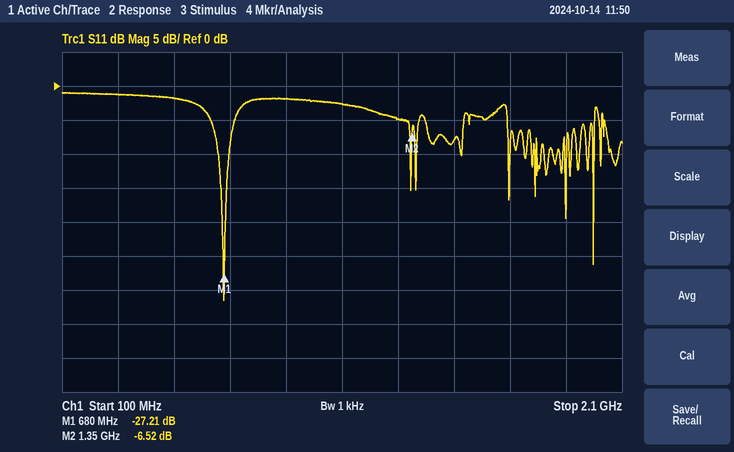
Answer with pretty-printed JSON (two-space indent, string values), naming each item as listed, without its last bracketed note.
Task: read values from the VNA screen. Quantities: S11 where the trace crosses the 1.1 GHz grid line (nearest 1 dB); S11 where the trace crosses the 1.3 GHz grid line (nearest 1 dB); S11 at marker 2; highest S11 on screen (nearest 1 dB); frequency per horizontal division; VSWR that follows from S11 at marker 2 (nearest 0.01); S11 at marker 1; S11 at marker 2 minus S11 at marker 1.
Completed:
{
  "S11 where the trace crosses the 1.1 GHz grid line": "-3 dB",
  "S11 where the trace crosses the 1.3 GHz grid line": "-5 dB",
  "S11 at marker 2": "-6.52 dB",
  "highest S11 on screen": "-1 dB",
  "frequency per horizontal division": "200 MHz",
  "VSWR that follows from S11 at marker 2": "2.79",
  "S11 at marker 1": "-27.21 dB",
  "S11 at marker 2 minus S11 at marker 1": "20.69 dB"
}
